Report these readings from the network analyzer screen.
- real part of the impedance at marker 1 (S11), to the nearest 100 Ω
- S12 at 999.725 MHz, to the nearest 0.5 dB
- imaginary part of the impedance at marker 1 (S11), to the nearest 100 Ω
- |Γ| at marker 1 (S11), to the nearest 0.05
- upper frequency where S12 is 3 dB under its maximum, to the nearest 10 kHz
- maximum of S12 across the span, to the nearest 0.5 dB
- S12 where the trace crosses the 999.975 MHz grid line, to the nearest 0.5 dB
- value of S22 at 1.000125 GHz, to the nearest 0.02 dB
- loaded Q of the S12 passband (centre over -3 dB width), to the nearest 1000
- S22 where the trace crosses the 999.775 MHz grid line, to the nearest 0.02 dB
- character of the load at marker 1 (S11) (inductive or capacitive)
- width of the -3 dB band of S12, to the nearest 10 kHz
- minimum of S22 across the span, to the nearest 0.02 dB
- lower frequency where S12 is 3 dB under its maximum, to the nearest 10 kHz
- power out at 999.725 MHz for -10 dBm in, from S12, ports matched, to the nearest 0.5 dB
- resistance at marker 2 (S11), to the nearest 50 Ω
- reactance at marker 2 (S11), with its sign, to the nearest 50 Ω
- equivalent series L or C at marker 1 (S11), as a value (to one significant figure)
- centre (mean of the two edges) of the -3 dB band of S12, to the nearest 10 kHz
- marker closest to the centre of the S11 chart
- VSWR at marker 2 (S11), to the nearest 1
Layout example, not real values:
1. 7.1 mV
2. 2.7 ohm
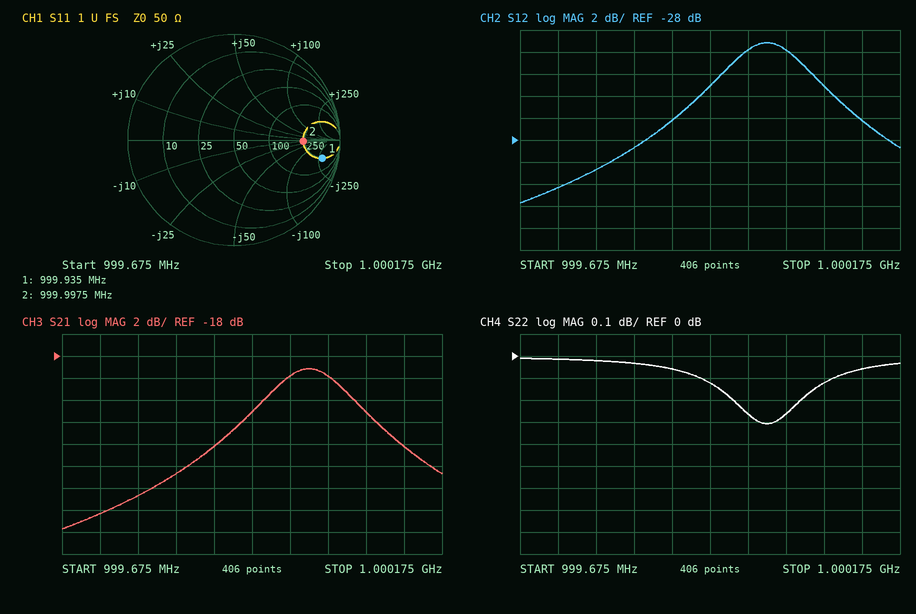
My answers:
1. 200 Ω
2. -32.5 dB
3. -300 Ω
4. 0.85
5. 1.00006 GHz
6. -19.0 dB
7. -20.0 dB
8. -0.06 dB
9. 8000
10. -0.02 dB
11. capacitive
12. 120 kHz
13. -0.30 dB
14. 999.94 MHz
15. -42.5 dBm
16. 250 Ω
17. 0 Ω
18. 500 fF
19. 1.00000 GHz
20. marker 2
21. 5
